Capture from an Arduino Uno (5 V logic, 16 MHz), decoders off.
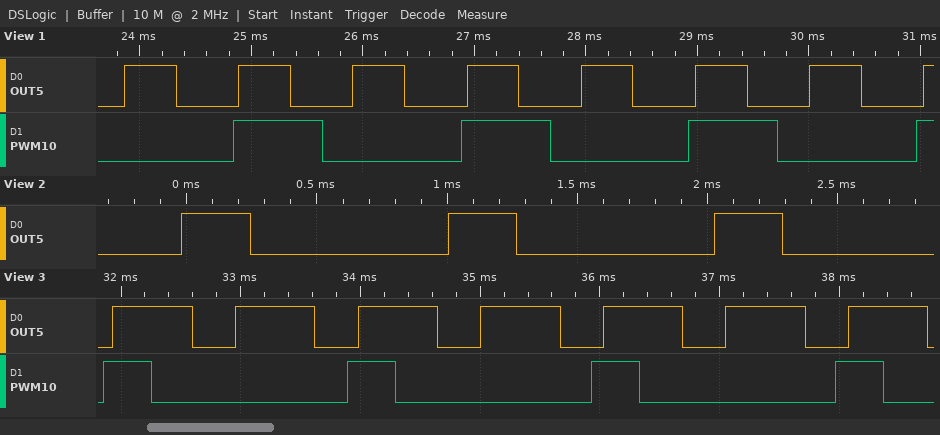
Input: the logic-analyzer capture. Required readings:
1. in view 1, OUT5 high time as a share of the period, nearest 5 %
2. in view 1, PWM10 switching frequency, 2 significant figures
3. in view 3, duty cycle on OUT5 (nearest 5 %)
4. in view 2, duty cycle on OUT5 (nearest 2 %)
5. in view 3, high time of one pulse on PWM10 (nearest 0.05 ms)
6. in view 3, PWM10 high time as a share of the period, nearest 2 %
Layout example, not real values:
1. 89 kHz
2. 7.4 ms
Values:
1. 45 %
2. 490 Hz
3. 65 %
4. 26 %
5. 0.40 ms
6. 20 %
